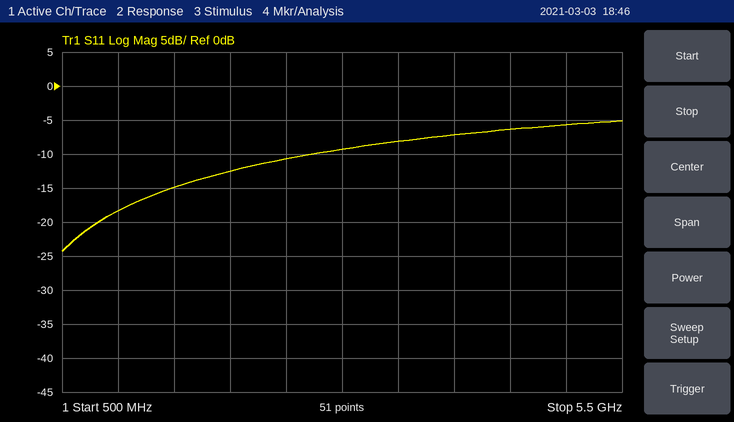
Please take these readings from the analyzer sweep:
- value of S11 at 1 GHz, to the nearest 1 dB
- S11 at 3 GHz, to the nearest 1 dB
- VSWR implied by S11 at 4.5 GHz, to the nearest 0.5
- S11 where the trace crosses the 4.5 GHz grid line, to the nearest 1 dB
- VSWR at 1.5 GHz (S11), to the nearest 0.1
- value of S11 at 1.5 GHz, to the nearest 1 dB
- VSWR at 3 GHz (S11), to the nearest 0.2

-18 dB
-9 dB
3.0
-6 dB
1.4
-15 dB
2.0
